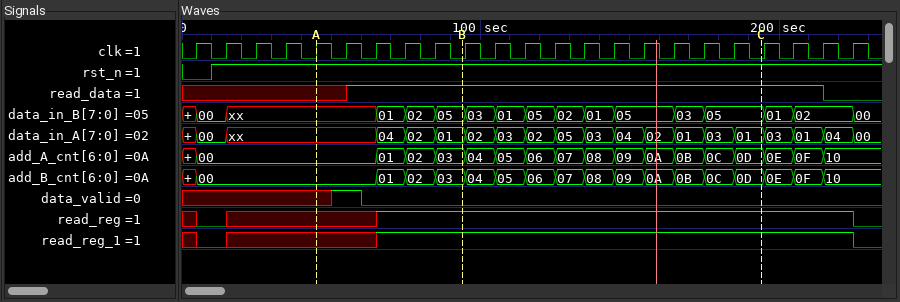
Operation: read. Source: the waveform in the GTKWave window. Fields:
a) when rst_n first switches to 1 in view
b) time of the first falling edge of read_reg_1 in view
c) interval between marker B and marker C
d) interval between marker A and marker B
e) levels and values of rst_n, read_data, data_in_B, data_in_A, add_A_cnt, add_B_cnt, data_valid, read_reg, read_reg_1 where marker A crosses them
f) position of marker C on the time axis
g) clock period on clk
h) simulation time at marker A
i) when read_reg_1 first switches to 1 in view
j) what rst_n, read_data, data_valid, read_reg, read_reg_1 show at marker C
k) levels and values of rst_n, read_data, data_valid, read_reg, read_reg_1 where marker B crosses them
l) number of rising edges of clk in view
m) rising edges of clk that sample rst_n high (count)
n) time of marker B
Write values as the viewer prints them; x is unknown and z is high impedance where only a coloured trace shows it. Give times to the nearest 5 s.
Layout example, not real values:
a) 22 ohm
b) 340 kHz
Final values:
a) 10 s
b) 225 s
c) 100 s
d) 50 s
e) rst_n=1, read_data=x, data_in_B=xx, data_in_A=xx, add_A_cnt=00, add_B_cnt=00, data_valid=x, read_reg=x, read_reg_1=x
f) 195 s
g) 10 s
h) 45 s
i) 65 s
j) rst_n=1, read_data=1, data_valid=0, read_reg=1, read_reg_1=1
k) rst_n=1, read_data=1, data_valid=0, read_reg=1, read_reg_1=1
l) 23
m) 22
n) 95 s
